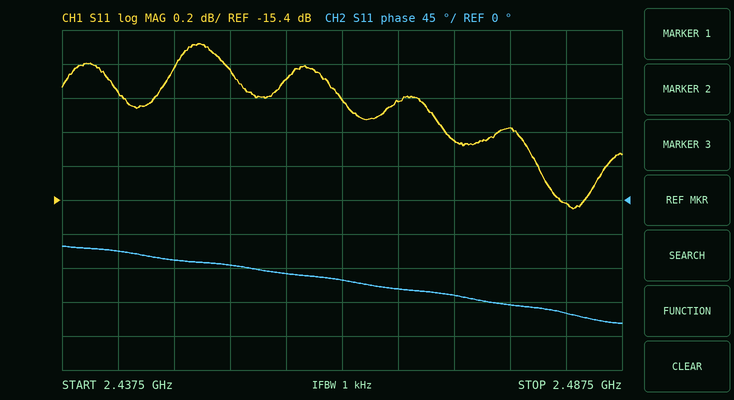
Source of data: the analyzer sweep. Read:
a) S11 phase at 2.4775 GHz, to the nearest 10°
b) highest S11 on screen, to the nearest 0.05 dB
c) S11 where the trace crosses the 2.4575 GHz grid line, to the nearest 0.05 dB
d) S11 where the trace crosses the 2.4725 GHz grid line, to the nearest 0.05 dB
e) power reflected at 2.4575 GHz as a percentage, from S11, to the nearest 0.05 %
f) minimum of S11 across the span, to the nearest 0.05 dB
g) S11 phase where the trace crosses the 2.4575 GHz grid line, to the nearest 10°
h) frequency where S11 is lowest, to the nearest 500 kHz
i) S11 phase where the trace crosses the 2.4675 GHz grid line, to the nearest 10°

-140°
-14.50 dB
-14.70 dB
-15.05 dB
3.40 %
-15.45 dB
-100°
2.4830 GHz
-120°
